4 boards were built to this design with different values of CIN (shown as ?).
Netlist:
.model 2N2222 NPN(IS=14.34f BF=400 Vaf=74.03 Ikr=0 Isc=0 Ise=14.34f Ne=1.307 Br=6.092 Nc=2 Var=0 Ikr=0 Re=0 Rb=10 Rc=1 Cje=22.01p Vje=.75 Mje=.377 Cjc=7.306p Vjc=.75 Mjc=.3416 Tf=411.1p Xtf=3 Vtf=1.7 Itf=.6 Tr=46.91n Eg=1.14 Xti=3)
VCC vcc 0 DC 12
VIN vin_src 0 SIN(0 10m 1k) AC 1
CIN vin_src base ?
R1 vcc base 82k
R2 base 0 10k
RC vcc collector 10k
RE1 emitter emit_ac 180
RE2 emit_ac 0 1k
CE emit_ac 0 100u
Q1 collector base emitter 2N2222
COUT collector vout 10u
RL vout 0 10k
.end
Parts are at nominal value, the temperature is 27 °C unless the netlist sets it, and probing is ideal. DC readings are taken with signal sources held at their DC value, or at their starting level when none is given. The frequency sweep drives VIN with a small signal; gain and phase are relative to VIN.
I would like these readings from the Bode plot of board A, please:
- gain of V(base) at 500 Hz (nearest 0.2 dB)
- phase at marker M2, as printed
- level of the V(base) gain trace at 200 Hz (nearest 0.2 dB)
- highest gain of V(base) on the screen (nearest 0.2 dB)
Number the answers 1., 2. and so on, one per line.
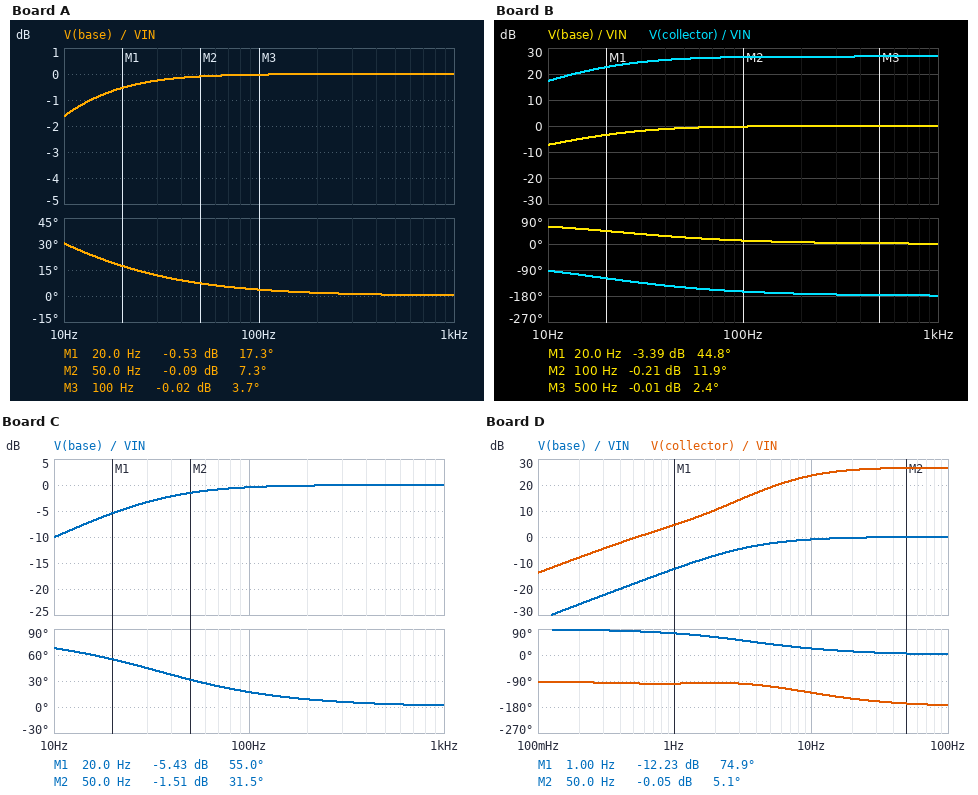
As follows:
1. 0 dB
2. 7.3 deg
3. 0 dB
4. 0 dB
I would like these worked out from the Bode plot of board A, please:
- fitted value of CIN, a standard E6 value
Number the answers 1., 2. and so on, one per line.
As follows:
1. 3.3 µF
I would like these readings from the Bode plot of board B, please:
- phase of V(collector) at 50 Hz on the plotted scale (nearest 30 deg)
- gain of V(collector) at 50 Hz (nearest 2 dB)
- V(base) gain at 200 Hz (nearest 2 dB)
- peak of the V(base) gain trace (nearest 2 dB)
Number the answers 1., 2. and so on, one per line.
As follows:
1. -150 deg
2. 26 dB
3. 0 dB
4. 0 dB
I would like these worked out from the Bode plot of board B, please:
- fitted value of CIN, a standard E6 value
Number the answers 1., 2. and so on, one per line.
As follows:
1. 1 µF
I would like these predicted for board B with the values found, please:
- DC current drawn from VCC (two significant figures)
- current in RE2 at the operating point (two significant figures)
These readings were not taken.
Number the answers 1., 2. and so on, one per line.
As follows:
1. 680 µA
2. 550 µA
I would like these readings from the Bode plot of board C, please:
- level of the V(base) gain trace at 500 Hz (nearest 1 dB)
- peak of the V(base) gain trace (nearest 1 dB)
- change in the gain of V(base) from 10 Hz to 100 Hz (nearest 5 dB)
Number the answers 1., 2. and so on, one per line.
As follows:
1. 0 dB
2. 0 dB
3. 10 dB
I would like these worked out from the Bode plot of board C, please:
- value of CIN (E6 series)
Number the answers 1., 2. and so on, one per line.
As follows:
1. 680 nF
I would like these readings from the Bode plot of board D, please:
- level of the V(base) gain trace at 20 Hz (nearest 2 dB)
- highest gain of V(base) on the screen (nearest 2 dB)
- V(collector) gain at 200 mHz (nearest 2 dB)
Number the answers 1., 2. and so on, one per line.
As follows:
1. 0 dB
2. 0 dB
3. -8 dB
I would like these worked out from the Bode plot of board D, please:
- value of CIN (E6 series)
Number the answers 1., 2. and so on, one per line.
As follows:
1. 4.7 µF
